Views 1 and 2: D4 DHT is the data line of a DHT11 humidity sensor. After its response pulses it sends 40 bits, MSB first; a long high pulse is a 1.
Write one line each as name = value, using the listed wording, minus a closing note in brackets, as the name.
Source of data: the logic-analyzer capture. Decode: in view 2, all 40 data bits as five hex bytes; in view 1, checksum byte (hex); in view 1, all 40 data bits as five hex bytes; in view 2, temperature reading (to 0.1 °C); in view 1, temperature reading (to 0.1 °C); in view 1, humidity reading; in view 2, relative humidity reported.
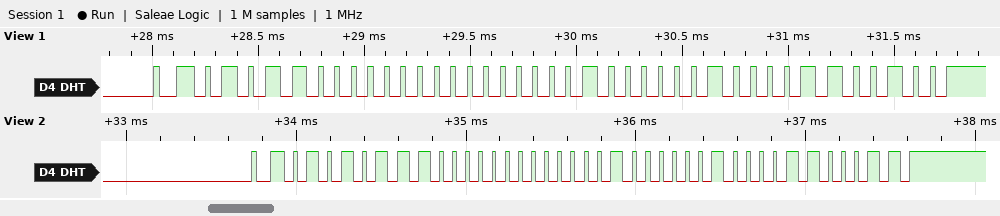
in view 2, all 40 data bits as five hex bytes = 57 00 04 08 63
in view 1, checksum byte = 0x64
in view 1, all 40 data bits as five hex bytes = 58 00 04 08 64
in view 2, temperature reading = 4.8 °C
in view 1, temperature reading = 4.8 °C
in view 1, humidity reading = 88 %
in view 2, relative humidity reported = 87 %
